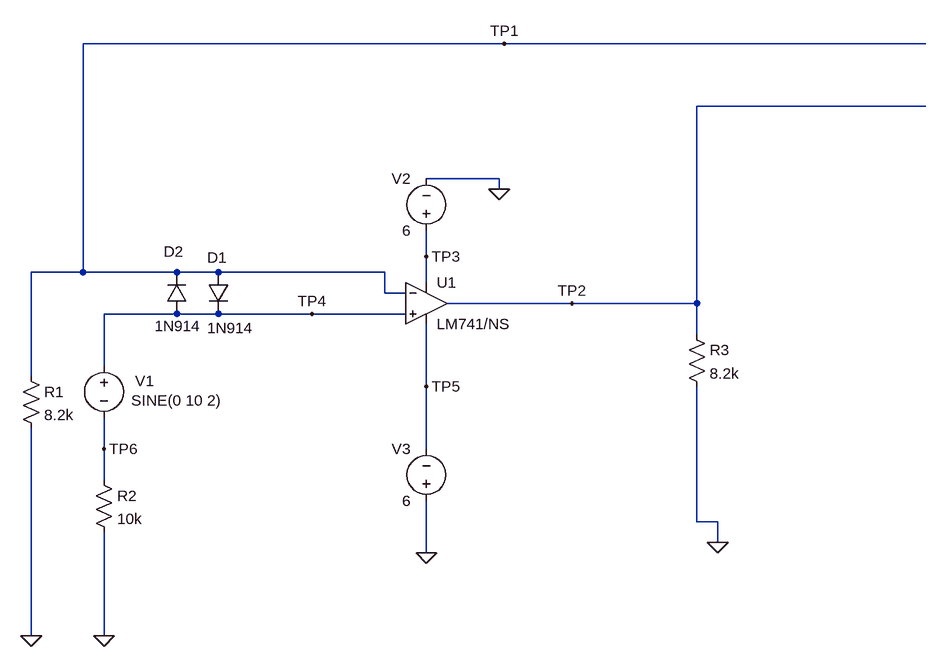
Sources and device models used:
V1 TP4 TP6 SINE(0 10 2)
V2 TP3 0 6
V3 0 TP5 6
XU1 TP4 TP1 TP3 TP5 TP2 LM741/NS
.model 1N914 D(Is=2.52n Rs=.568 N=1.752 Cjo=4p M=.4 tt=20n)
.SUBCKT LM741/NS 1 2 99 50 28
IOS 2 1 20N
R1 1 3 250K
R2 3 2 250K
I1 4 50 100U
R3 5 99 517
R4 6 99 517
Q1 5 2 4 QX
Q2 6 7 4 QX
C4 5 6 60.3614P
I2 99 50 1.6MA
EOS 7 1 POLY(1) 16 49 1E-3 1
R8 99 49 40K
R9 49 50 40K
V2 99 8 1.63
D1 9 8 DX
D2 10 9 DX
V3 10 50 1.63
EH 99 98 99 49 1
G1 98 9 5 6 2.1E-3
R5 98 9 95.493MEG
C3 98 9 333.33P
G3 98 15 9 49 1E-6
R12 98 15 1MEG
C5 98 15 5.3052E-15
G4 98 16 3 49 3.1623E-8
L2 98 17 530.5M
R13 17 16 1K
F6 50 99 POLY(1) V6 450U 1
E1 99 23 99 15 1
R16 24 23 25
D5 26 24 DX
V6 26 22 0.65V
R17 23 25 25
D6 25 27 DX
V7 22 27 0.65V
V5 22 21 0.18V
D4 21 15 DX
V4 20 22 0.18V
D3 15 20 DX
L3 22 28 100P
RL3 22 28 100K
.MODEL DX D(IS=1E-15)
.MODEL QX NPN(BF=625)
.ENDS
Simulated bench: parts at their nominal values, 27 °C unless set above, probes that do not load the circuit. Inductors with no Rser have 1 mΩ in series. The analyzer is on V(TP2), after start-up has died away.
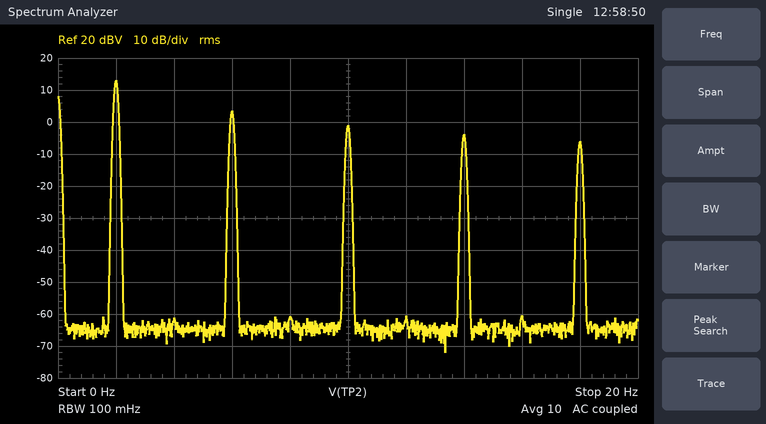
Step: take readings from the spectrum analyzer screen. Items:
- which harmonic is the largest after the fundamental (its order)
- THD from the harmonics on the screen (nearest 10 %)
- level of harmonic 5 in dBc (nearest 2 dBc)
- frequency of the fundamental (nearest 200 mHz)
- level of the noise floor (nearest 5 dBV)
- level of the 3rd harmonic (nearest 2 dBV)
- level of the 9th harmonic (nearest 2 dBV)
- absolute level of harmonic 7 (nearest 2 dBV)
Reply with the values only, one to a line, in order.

3
40 %
-14 dBc
2.0 Hz
-65 dBV
4 dBV
-6 dBV
-4 dBV
